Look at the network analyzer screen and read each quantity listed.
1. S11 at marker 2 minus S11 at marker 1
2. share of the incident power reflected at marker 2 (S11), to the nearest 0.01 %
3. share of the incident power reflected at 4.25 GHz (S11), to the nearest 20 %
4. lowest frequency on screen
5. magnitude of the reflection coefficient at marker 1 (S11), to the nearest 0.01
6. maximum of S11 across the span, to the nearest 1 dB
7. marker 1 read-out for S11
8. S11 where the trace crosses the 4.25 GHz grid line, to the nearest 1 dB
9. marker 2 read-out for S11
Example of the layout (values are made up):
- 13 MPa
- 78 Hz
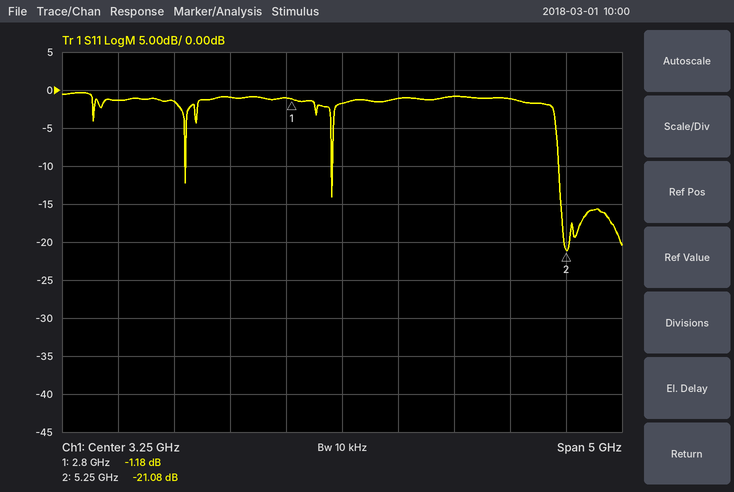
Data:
- -19.90 dB
- 0.78 %
- 80 %
- 750 MHz
- 0.87
- 0 dB
- -1.18 dB
- -1 dB
- -21.08 dB
